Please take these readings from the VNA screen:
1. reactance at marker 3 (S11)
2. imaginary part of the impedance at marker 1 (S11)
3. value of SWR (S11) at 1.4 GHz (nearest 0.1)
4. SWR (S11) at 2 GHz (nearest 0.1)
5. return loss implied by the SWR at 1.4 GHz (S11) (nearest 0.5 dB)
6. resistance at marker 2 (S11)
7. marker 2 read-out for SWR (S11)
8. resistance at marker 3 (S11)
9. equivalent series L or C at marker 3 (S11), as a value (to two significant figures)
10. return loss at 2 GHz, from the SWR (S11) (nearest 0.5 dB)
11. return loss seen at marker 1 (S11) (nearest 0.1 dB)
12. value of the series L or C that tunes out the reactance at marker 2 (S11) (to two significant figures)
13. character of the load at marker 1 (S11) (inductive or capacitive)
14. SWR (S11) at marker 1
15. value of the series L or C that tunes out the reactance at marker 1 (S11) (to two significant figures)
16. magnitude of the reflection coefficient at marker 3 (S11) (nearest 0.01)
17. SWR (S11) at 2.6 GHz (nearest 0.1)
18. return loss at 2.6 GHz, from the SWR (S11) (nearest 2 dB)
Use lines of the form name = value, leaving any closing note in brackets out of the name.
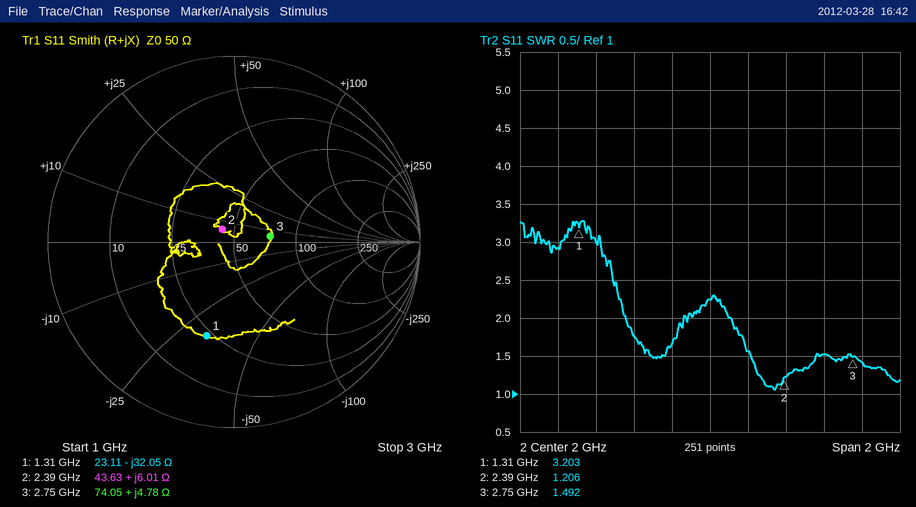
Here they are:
reactance at marker 3 = +4.78 Ω
imaginary part of the impedance at marker 1 = -32.05 Ω
value of SWR (S11) at 1.4 GHz = 3.0
SWR (S11) at 2 GHz = 2.2
return loss implied by the SWR at 1.4 GHz (S11) = 6.0 dB
resistance at marker 2 = 43.63 Ω
marker 2 read-out for SWR = 1.206
resistance at marker 3 = 74.05 Ω
equivalent series L or C at marker 3 (S11), as a value = 280 pH
return loss at 2 GHz, from the SWR (S11) = 8.5 dB
return loss seen at marker 1 (S11) = 5.6 dB
value of the series L or C that tunes out the reactance at marker 2 (S11) = 11 pF
character of the load at marker 1 (S11) = capacitive
SWR (S11) at marker 1 = 3.203
value of the series L or C that tunes out the reactance at marker 1 (S11) = 3.9 nH
magnitude of the reflection coefficient at marker 3 (S11) = 0.20
SWR (S11) at 2.6 GHz = 1.5
return loss at 2.6 GHz, from the SWR (S11) = 14 dB
